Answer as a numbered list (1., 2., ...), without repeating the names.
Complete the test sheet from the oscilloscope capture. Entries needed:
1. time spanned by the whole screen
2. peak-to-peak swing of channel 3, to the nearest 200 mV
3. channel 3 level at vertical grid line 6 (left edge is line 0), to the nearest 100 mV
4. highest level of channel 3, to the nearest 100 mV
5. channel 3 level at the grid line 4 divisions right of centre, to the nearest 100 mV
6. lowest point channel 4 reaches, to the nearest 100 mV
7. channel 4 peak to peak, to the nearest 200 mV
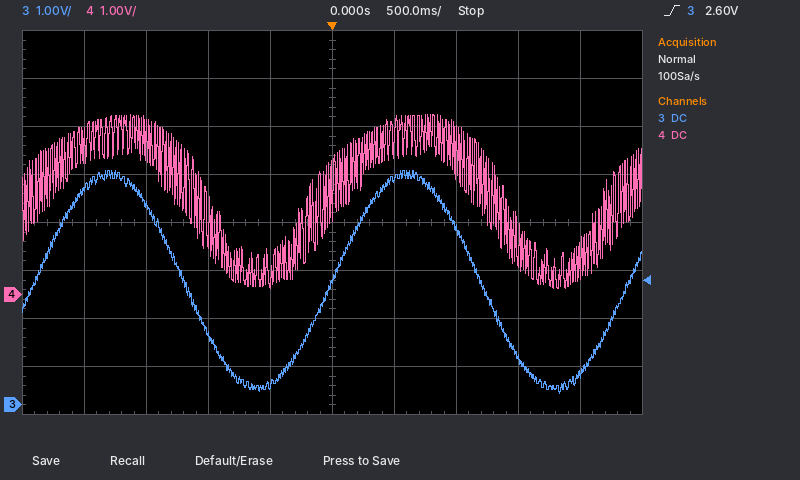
1. 5 s
2. 4.6 V
3. 4.7 V
4. 4.9 V
5. 700 mV
6. 100 mV
7. 3.6 V
